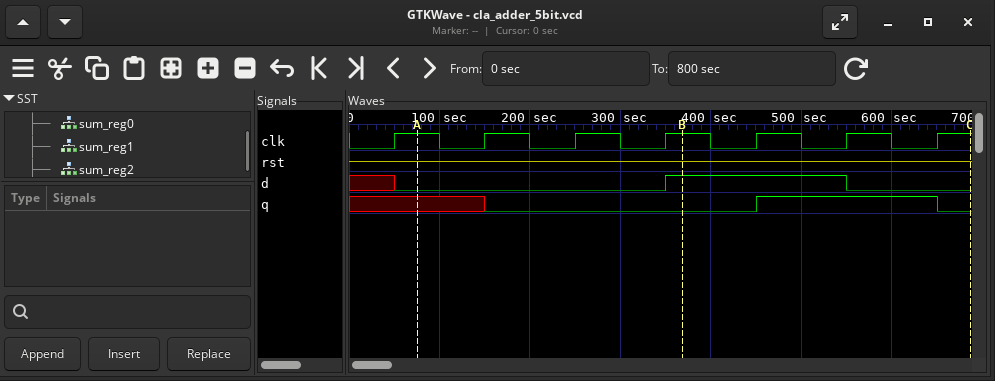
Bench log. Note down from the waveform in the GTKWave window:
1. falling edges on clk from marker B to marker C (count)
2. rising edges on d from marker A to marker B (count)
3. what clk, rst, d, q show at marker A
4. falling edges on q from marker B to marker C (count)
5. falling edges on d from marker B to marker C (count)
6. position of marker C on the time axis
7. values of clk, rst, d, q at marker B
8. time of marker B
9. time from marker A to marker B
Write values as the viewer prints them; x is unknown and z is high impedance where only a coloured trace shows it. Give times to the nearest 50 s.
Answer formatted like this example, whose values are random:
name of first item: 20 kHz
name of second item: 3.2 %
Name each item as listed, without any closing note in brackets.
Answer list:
falling edges on clk from marker B to marker C: 3
rising edges on d from marker A to marker B: 1
what clk, rst, d, q show at marker A: clk=1, rst=z, d=0, q=x
falling edges on q from marker B to marker C: 1
falling edges on d from marker B to marker C: 1
position of marker C on the time axis: 700 s
values of clk, rst, d, q at marker B: clk=1, rst=z, d=1, q=0
time of marker B: 350 s
time from marker A to marker B: 300 s
